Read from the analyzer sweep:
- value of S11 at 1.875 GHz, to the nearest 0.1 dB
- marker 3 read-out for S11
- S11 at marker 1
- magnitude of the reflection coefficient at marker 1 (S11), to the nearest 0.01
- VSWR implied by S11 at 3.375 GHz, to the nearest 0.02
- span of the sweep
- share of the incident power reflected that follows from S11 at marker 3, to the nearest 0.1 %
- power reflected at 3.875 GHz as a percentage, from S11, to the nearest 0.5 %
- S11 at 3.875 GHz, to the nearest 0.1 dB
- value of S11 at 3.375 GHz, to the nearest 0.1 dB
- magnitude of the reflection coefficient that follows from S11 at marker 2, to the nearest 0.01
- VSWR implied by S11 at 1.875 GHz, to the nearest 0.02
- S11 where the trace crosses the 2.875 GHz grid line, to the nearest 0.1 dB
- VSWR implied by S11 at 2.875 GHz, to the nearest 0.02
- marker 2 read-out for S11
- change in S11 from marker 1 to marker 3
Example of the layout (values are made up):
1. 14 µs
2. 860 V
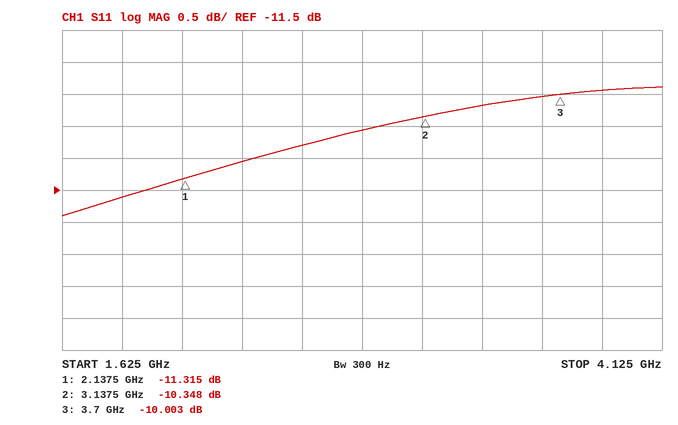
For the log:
1. -11.6 dB
2. -10.003 dB
3. -11.315 dB
4. 0.27
5. 1.90
6. 2.5 GHz
7. 10.0 %
8. 10.0 %
9. -9.9 dB
10. -10.2 dB
11. 0.30
12. 1.72
13. -10.6 dB
14. 1.84
15. -10.348 dB
16. 1.312 dB
